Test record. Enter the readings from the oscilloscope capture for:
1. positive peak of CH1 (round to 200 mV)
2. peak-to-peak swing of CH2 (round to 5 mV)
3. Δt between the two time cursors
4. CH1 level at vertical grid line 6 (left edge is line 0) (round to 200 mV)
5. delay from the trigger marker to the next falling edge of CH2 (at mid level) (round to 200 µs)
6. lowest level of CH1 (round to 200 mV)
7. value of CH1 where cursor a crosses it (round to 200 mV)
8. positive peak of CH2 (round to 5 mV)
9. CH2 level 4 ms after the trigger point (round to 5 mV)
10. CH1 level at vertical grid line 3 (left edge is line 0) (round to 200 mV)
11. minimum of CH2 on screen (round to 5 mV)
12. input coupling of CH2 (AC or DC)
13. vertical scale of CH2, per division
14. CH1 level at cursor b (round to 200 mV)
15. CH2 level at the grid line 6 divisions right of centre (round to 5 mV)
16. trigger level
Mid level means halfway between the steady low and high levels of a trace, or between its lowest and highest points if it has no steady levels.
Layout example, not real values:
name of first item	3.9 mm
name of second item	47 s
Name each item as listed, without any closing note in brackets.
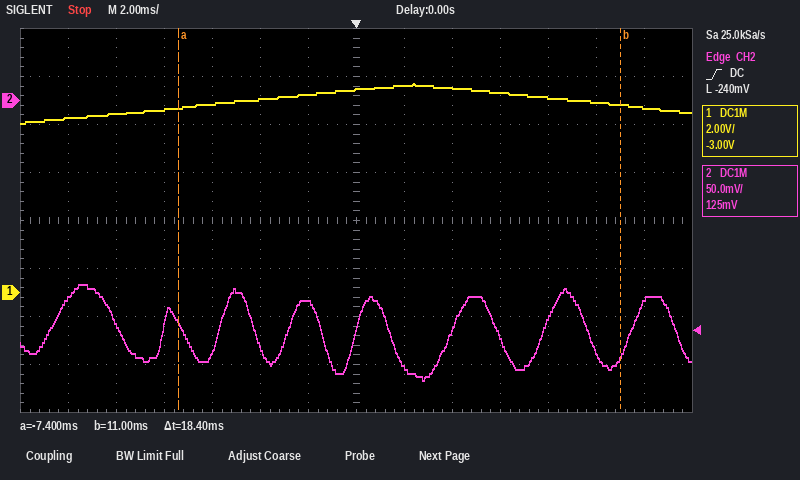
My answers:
positive peak of CH1	8.8 V
peak-to-peak swing of CH2	100 mV
Δt between the two time cursors	18.4 ms
CH1 level at vertical grid line 6 (left edge is line 0)	8.2 V
delay from the trigger marker to the next falling edge of CH2 (at mid level)	1.4 ms
lowest level of CH1	7.0 V
value of CH1 where cursor a crosses it	7.6 V
positive peak of CH2	-190 mV
CH2 level 4 ms after the trigger point	-240 mV
CH1 level at vertical grid line 3 (left edge is line 0)	7.6 V
minimum of CH2 on screen	-290 mV
input coupling of CH2	DC
vertical scale of CH2, per division	50 mV
CH1 level at cursor b	7.8 V
CH2 level at the grid line 6 divisions right of centre	-210 mV
trigger level	-240 mV
